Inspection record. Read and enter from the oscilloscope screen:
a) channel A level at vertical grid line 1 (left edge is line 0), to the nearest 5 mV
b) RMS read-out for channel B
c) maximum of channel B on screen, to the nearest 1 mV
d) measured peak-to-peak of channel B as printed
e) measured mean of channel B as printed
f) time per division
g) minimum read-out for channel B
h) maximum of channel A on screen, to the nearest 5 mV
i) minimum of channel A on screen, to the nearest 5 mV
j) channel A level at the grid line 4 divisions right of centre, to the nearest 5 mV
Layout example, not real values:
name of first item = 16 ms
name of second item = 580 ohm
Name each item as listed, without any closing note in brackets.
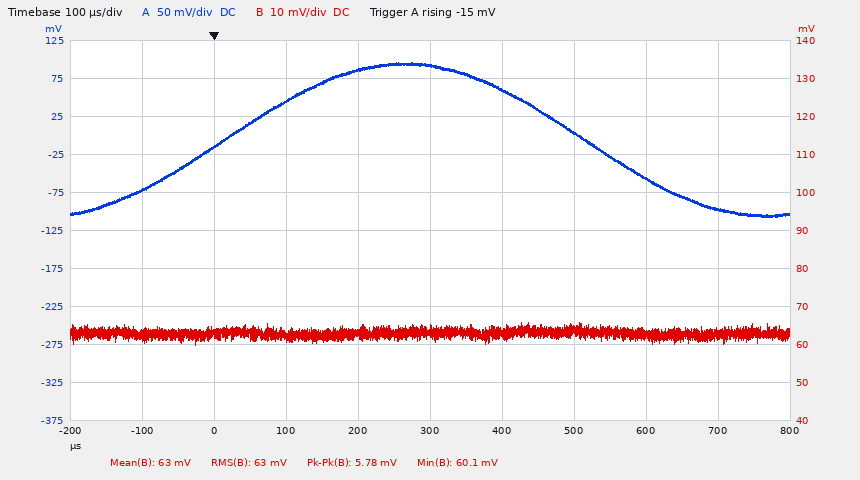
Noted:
channel A level at vertical grid line 1 (left edge is line 0), to the nearest 5 mV = -70 mV
RMS read-out for channel B = 63 mV
maximum of channel B on screen, to the nearest 1 mV = 66 mV
measured peak-to-peak of channel B as printed = 5.78 mV
measured mean of channel B as printed = 63 mV
time per division = 100 µs
minimum read-out for channel B = 60.1 mV
maximum of channel A on screen, to the nearest 5 mV = 95 mV
minimum of channel A on screen, to the nearest 5 mV = -105 mV
channel A level at the grid line 4 divisions right of centre, to the nearest 5 mV = -95 mV
